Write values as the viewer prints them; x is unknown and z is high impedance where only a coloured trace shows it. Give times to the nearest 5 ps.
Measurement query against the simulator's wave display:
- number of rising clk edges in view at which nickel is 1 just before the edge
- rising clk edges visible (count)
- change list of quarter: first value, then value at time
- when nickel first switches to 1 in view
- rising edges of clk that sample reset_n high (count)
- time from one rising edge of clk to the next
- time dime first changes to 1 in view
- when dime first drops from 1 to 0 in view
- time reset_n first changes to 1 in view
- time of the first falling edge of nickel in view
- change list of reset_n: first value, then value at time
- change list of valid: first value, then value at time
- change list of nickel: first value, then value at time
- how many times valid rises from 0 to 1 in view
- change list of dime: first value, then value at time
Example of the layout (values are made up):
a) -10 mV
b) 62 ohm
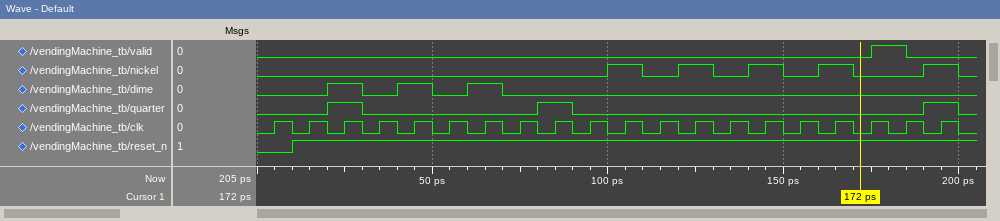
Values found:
a) 5
b) 20
c) 0, 1 at 20 ps, 0 at 30 ps, 1 at 80 ps, 0 at 90 ps, 1 at 190 ps, 0 at 200 ps
d) 100 ps
e) 19
f) 10 ps
g) 20 ps
h) 30 ps
i) 10 ps
j) 110 ps
k) 0, 1 at 10 ps
l) 0, 1 at 175 ps, 0 at 185 ps
m) 0, 1 at 100 ps, 0 at 110 ps, 1 at 120 ps, 0 at 130 ps, 1 at 140 ps, 0 at 150 ps, 1 at 160 ps, 0 at 170 ps, 1 at 190 ps, 0 at 200 ps
n) 1
o) 0, 1 at 20 ps, 0 at 30 ps, 1 at 40 ps, 0 at 50 ps, 1 at 60 ps, 0 at 70 ps
